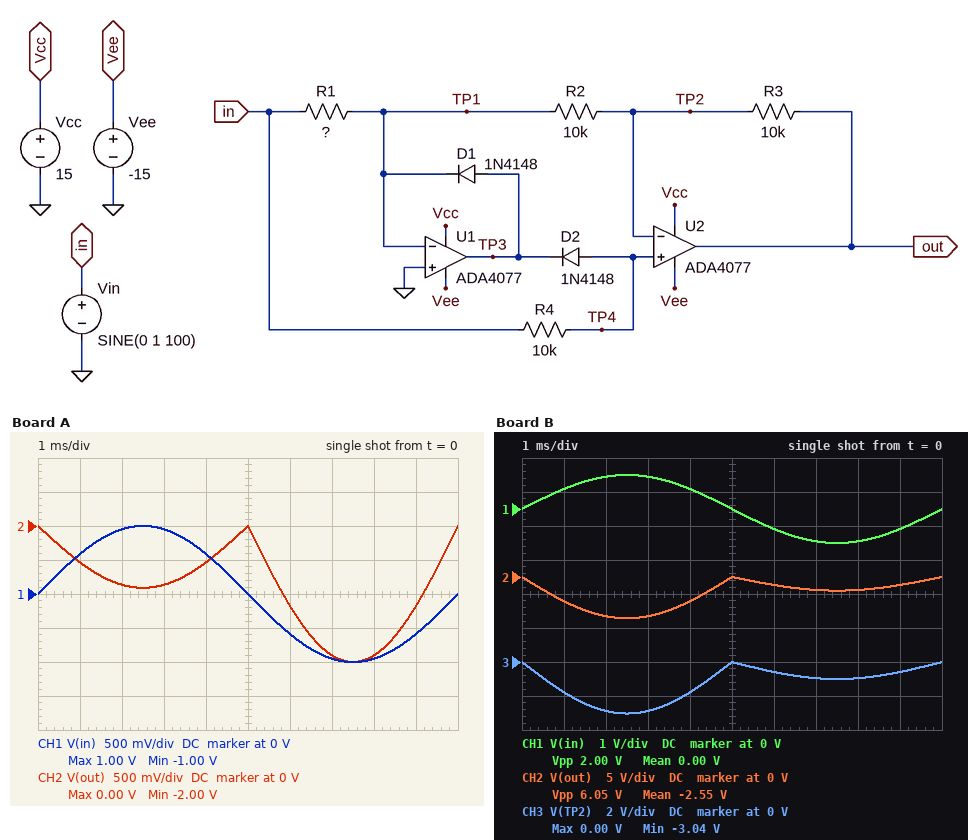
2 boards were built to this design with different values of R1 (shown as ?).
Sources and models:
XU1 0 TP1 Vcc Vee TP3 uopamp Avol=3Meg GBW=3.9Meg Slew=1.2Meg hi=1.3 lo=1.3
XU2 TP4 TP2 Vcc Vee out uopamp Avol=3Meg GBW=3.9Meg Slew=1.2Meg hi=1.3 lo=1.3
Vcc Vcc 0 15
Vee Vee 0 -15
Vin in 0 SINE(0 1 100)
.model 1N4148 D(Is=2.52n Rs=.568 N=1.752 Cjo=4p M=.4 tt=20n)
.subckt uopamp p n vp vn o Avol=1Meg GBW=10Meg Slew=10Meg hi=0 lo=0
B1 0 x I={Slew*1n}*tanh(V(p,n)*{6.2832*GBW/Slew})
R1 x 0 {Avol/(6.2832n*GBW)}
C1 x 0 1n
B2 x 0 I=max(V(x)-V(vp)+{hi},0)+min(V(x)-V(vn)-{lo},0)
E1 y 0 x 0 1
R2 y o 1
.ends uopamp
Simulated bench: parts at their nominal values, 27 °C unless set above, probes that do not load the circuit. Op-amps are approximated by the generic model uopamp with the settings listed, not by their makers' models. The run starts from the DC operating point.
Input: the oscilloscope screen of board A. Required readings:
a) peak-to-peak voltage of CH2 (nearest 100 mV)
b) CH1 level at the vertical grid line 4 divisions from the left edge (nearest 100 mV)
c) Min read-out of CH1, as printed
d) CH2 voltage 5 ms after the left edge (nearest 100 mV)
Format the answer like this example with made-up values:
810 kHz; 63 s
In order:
2.0 V; 600 mV; -1.00 V; 0 V
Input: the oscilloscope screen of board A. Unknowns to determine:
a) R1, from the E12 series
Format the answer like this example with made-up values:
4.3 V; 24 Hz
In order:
22 kΩ
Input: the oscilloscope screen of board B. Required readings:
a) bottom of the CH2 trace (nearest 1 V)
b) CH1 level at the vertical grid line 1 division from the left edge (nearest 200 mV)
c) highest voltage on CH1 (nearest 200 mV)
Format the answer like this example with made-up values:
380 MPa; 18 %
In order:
-6 V; 600 mV; 1.0 V
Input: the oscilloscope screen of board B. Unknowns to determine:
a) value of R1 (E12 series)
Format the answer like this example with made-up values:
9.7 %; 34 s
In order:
3.3 kΩ
